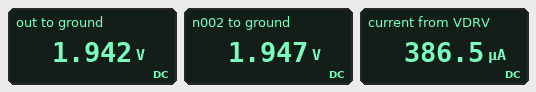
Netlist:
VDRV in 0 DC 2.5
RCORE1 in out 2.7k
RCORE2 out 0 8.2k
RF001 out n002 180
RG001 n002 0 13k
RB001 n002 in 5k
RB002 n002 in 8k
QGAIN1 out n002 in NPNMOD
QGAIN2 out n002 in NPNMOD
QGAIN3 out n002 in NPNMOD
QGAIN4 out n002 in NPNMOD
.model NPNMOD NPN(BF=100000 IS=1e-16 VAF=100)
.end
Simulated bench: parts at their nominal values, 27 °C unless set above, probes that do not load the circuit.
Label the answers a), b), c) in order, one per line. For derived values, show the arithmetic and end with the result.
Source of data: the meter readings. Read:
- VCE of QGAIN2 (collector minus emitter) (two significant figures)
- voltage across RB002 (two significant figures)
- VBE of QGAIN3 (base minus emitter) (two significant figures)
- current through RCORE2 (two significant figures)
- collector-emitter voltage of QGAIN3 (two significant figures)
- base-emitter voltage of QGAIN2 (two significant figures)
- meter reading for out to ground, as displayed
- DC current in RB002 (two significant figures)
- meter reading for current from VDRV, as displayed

a) 1.942 V - 2.5 V = -560 mV
b) 2.5 V - 1.947 V = 550 mV
c) 1.947 V - 2.5 V = -550 mV
d) (1.942 V) / 8.2 kΩ = 240 µA
e) 1.942 V - 2.5 V = -560 mV
f) 1.947 V - 2.5 V = -550 mV
g) 1.942 V
h) (2.5 V - 1.947 V) / 8 kΩ = 69 µA
i) 386.5 µA
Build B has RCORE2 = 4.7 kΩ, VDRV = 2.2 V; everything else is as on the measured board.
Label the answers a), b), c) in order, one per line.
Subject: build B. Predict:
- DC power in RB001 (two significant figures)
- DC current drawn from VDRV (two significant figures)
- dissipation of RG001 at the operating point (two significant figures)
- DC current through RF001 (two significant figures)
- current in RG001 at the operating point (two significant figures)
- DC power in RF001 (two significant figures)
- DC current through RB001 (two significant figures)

a) 81 µW
b) 450 µA
c) 190 µW
d) 87 µA
e) 120 µA
f) 1.4 µW
g) 130 µA
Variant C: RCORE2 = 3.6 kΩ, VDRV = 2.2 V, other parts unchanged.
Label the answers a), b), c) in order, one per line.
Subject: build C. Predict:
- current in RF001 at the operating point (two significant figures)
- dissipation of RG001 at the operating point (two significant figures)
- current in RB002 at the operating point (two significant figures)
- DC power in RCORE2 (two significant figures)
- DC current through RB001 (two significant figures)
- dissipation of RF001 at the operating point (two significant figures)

a) 120 µA
b) 170 µW
c) 91 µA
d) 580 µW
e) 150 µA
f) 2.8 µW
